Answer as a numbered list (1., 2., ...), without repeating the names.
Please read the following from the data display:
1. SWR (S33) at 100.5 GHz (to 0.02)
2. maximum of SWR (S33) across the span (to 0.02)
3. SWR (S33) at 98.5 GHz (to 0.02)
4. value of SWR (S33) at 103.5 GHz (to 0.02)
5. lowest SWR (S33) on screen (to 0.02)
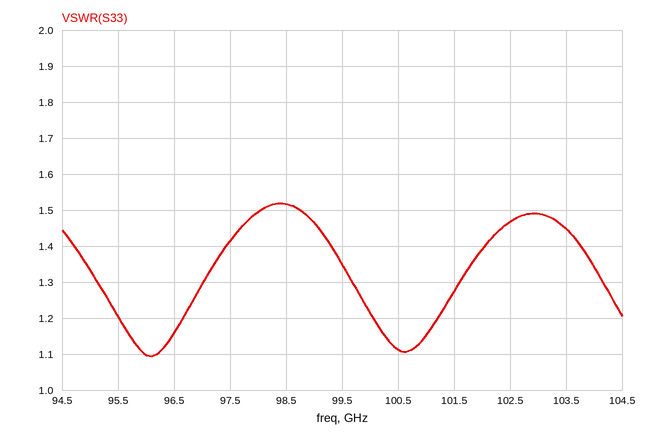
1. 1.12
2. 1.52
3. 1.52
4. 1.44
5. 1.10
